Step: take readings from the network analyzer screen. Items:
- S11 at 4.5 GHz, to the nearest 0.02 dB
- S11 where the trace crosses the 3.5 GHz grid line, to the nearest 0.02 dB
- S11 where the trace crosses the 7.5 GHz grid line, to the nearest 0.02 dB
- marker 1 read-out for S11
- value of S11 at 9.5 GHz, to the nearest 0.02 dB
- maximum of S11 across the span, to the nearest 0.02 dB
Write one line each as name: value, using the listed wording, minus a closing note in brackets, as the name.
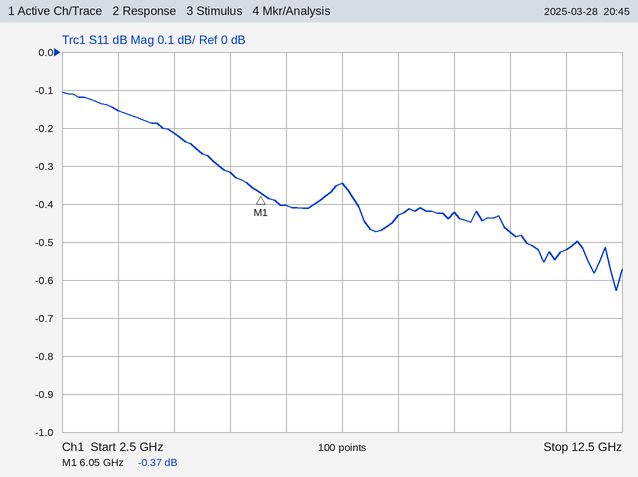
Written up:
S11 at 4.5 GHz, to the nearest 0.02 dB: -0.22 dB
S11 where the trace crosses the 3.5 GHz grid line, to the nearest 0.02 dB: -0.16 dB
S11 where the trace crosses the 7.5 GHz grid line, to the nearest 0.02 dB: -0.34 dB
marker 1 read-out for S11: -0.37 dB
value of S11 at 9.5 GHz, to the nearest 0.02 dB: -0.42 dB
maximum of S11 across the span, to the nearest 0.02 dB: -0.10 dB
